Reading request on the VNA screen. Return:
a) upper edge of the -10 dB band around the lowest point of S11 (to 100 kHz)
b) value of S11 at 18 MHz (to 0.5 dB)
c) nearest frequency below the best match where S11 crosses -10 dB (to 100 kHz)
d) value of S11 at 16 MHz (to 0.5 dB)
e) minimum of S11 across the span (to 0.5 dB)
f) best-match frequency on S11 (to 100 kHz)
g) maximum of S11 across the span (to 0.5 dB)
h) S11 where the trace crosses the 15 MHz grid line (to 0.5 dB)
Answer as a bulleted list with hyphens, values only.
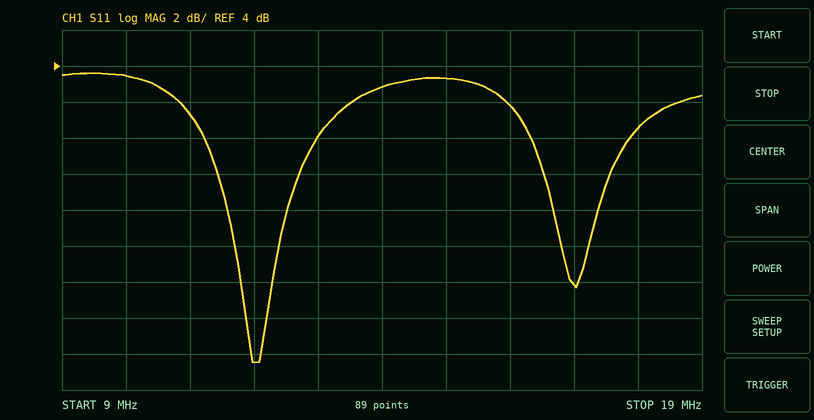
- 12.2 MHz
- 0.5 dB
- 11.9 MHz
- 2.0 dB
- -12.5 dB
- 12.0 MHz
- 3.5 dB
- 3.5 dB
